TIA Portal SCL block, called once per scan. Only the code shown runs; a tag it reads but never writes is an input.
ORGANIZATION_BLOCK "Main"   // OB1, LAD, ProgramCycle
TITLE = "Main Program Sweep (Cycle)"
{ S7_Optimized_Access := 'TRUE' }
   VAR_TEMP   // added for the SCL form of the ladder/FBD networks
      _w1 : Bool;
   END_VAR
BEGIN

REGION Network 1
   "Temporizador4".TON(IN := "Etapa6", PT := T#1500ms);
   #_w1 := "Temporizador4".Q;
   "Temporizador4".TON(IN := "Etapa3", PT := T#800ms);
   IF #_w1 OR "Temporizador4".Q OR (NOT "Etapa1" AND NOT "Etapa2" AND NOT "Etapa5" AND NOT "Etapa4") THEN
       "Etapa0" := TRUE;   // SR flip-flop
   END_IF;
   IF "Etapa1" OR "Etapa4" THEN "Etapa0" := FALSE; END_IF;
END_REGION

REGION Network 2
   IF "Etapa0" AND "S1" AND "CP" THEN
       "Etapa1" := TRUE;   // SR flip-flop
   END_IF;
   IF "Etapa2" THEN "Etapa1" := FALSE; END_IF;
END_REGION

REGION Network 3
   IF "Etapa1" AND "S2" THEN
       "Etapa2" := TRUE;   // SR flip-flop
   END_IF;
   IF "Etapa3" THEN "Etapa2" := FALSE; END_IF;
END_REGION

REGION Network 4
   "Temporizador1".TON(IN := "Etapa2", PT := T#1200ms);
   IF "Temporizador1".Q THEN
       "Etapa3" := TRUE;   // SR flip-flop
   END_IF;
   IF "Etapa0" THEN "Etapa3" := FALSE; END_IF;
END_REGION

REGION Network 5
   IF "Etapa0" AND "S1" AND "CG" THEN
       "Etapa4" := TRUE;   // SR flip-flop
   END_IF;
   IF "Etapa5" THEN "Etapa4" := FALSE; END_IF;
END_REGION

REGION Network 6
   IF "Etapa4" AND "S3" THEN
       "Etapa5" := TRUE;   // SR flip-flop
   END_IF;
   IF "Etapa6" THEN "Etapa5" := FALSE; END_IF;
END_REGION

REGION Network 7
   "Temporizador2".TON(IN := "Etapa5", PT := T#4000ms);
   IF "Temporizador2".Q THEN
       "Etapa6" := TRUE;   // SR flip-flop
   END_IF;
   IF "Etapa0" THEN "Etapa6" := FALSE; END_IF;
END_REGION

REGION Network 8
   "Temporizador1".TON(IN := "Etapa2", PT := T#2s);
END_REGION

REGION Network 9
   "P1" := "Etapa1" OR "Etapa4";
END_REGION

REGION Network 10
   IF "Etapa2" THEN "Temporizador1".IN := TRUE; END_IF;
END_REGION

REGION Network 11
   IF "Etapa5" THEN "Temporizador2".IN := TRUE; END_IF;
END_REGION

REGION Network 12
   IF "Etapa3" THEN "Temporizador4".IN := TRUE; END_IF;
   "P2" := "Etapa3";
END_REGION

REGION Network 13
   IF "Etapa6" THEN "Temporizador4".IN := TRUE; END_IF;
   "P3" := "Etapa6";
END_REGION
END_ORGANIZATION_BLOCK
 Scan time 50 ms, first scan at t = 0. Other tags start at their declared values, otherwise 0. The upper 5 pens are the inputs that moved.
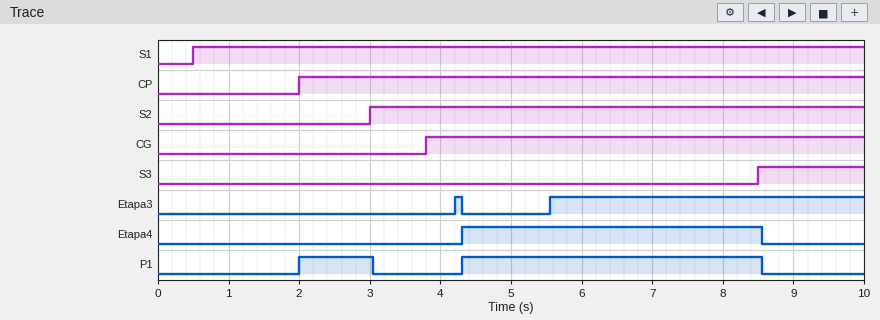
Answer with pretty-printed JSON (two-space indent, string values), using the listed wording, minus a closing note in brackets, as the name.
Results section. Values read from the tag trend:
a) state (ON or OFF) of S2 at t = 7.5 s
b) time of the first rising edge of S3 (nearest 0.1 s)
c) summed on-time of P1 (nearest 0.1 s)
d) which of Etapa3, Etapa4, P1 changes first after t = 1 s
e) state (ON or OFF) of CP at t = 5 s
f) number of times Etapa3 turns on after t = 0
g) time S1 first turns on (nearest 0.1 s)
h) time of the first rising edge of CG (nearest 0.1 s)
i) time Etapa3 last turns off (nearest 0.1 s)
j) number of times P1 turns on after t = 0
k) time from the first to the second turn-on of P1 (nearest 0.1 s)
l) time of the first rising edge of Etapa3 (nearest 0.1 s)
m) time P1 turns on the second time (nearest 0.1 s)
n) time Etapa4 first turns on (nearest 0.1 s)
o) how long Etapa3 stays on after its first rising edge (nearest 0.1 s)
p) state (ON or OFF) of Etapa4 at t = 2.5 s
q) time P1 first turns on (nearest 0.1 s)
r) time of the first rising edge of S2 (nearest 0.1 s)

{
  "state (ON or OFF) of S2 at t = 7.5 s": "ON",
  "time of the first rising edge of S3": "8.5 s",
  "summed on-time of P1": "5.3 s",
  "which of Etapa3, Etapa4, P1 changes first after t = 1 s": "P1",
  "state (ON or OFF) of CP at t = 5 s": "ON",
  "number of times Etapa3 turns on after t = 0": "2",
  "time S1 first turns on": "0.5 s",
  "time of the first rising edge of CG": "3.8 s",
  "time Etapa3 last turns off": "4.3 s",
  "number of times P1 turns on after t = 0": "2",
  "time from the first to the second turn-on of P1": "2.3 s",
  "time of the first rising edge of Etapa3": "4.2 s",
  "time P1 turns on the second time": "4.3 s",
  "time Etapa4 first turns on": "4.3 s",
  "how long Etapa3 stays on after its first rising edge": "0.1 s",
  "state (ON or OFF) of Etapa4 at t = 2.5 s": "OFF",
  "time P1 first turns on": "2.0 s",
  "time of the first rising edge of S2": "3.0 s"
}
